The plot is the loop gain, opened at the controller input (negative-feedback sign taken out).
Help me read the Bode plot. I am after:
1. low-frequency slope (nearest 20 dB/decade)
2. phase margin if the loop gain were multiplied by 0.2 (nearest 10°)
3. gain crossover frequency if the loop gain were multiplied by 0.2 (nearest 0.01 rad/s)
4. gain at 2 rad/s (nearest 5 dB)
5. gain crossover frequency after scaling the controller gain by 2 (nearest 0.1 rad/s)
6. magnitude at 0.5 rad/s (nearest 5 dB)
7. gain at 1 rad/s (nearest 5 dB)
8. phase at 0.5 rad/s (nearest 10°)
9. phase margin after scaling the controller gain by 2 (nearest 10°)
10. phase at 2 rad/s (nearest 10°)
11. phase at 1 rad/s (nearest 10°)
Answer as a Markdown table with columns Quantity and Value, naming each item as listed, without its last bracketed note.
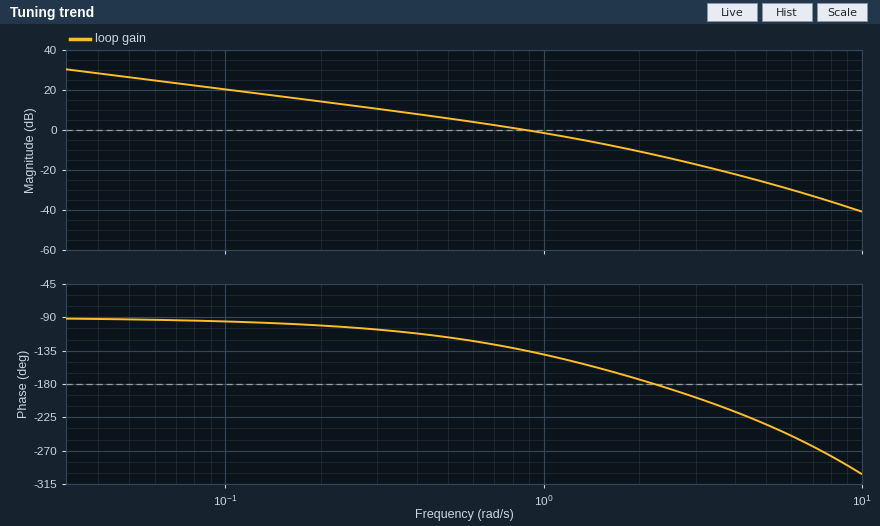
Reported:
| Quantity | Value |
|---|---|
| low-frequency slope | -20 dB/decade |
| phase margin if the loop gain were multiplied by 0.2 | 80° |
| gain crossover frequency if the loop gain were multiplied by 0.2 | 0.21 rad/s |
| gain at 2 rad/s | -10 dB |
| gain crossover frequency after scaling the controller gain by 2 | 1.4 rad/s |
| magnitude at 0.5 rad/s | 5 dB |
| gain at 1 rad/s | 0 dB |
| phase at 0.5 rad/s | -120° |
| phase margin after scaling the controller gain by 2 | 20° |
| phase at 2 rad/s | -170° |
| phase at 1 rad/s | -140° |
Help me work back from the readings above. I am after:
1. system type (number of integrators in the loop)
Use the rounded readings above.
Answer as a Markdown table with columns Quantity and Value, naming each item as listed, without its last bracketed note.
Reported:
| Quantity | Value |
|---|---|
| system type | 1 |
